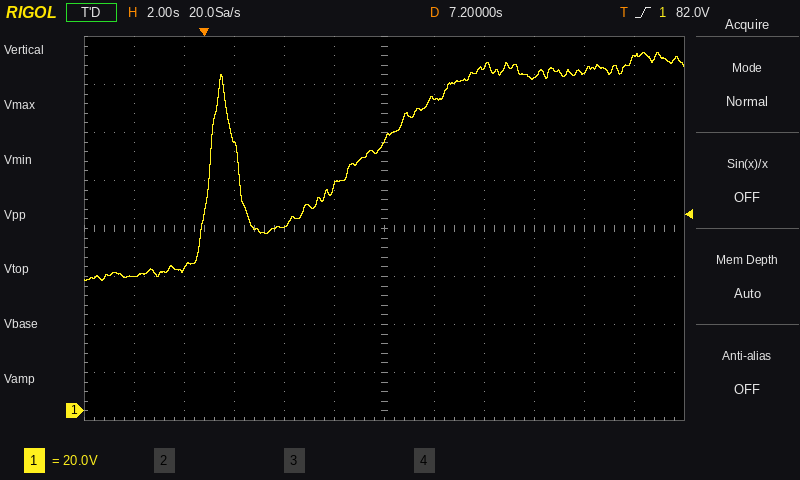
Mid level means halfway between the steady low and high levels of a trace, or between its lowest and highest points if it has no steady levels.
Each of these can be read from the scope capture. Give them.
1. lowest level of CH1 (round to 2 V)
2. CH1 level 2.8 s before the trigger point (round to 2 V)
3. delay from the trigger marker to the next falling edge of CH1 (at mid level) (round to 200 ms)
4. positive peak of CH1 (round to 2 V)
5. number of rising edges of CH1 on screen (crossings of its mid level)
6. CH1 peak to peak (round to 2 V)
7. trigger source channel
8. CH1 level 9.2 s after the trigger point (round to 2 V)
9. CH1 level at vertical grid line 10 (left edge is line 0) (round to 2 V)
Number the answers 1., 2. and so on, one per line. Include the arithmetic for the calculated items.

1. 54 V
2. 56 V
3. 1.4 s
4. 150 V
5. 2
6. 150 V − (54 V) = 96 V
7. CH1
8. 130 V
9. 142 V
